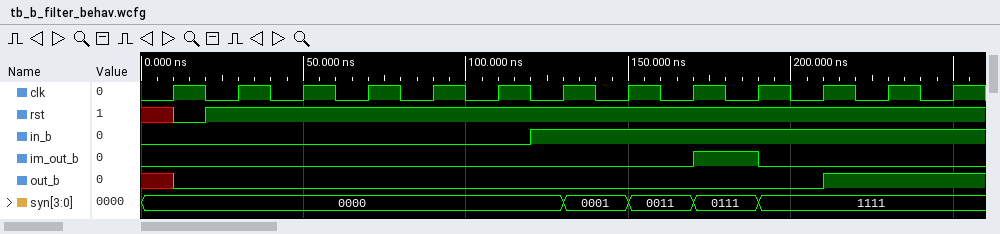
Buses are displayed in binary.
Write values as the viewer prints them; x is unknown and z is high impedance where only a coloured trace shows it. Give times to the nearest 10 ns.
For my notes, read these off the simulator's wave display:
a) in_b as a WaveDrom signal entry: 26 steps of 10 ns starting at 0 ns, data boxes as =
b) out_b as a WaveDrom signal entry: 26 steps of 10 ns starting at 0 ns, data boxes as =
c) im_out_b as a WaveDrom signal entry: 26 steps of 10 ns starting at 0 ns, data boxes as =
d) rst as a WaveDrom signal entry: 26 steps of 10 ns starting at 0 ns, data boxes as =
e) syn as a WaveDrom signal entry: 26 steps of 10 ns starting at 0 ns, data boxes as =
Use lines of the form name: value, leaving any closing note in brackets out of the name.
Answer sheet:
in_b as a WaveDrom signal entry: 26 steps of 10 ns starting at 0 ns, data boxes as =: {name: 'in_b', wave: '0...........1.............'}
out_b as a WaveDrom signal entry: 26 steps of 10 ns starting at 0 ns, data boxes as =: {name: 'out_b', wave: 'x0...................1....'}
im_out_b as a WaveDrom signal entry: 26 steps of 10 ns starting at 0 ns, data boxes as =: {name: 'im_out_b', wave: '0................1.0......'}
rst as a WaveDrom signal entry: 26 steps of 10 ns starting at 0 ns, data boxes as =: {name: 'rst', wave: 'x01.......................'}
syn as a WaveDrom signal entry: 26 steps of 10 ns starting at 0 ns, data boxes as =: {name: 'syn', wave: '=............=.=.=.=......', data: '0000 0001 0011 0111 1111'}
